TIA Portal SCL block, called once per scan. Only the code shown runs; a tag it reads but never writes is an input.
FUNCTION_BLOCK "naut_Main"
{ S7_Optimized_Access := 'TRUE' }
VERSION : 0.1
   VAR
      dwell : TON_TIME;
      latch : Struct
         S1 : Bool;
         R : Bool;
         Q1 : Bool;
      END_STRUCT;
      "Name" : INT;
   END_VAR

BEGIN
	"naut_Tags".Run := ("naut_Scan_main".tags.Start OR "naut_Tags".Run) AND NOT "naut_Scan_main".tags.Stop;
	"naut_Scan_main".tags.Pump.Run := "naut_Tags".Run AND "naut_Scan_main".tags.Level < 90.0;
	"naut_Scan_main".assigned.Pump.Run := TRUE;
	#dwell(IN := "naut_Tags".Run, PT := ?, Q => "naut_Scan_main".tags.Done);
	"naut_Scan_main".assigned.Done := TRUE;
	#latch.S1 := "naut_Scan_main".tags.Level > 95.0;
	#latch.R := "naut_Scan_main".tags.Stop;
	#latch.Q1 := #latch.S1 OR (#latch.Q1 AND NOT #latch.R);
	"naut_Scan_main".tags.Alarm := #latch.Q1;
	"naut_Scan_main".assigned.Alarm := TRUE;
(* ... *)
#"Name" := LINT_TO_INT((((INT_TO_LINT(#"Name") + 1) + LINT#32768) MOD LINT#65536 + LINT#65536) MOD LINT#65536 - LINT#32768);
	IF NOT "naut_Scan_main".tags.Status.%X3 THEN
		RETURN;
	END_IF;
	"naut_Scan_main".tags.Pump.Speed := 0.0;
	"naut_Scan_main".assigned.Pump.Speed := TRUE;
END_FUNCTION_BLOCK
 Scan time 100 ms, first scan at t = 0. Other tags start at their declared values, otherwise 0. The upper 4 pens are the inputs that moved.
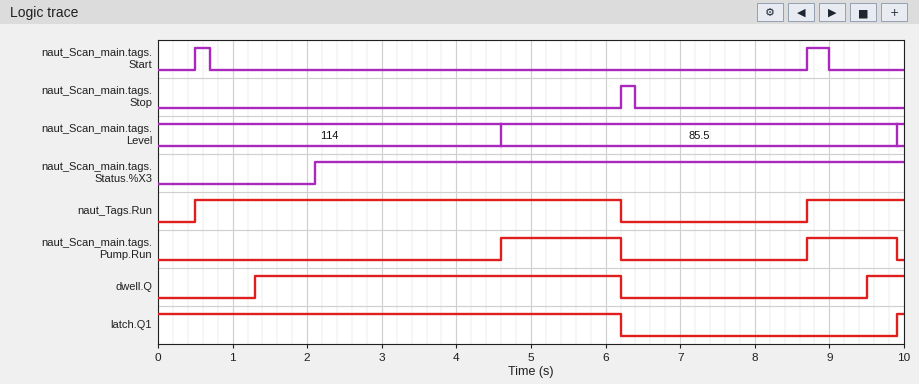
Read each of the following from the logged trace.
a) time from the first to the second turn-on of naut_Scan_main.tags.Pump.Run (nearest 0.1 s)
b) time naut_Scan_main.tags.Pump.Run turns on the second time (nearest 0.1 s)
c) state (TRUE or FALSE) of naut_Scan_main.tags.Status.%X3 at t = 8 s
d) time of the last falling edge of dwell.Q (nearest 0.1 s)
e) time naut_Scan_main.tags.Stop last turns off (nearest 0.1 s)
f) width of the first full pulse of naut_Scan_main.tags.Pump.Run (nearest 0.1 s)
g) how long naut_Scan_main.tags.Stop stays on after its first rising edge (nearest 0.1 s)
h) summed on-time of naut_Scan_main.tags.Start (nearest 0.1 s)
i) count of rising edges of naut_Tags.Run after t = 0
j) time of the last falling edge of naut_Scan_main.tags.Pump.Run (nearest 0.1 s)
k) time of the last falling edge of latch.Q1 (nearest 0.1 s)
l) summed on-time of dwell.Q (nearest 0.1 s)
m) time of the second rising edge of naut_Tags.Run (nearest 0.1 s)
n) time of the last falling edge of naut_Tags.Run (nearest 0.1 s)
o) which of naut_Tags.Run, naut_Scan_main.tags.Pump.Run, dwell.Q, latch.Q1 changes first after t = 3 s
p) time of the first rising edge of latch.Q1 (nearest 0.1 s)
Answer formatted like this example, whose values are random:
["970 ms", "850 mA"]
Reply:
["4.1 s", "8.7 s", "TRUE", "6.2 s", "6.4 s", "1.6 s", "0.2 s", "0.5 s", "2", "9.9 s", "6.2 s", "5.4 s", "8.7 s", "6.2 s", "naut_Scan_main.tags.Pump.Run", "9.9 s"]
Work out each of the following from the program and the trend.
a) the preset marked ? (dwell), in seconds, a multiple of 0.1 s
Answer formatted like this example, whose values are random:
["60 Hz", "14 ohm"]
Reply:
["0.8 s"]
